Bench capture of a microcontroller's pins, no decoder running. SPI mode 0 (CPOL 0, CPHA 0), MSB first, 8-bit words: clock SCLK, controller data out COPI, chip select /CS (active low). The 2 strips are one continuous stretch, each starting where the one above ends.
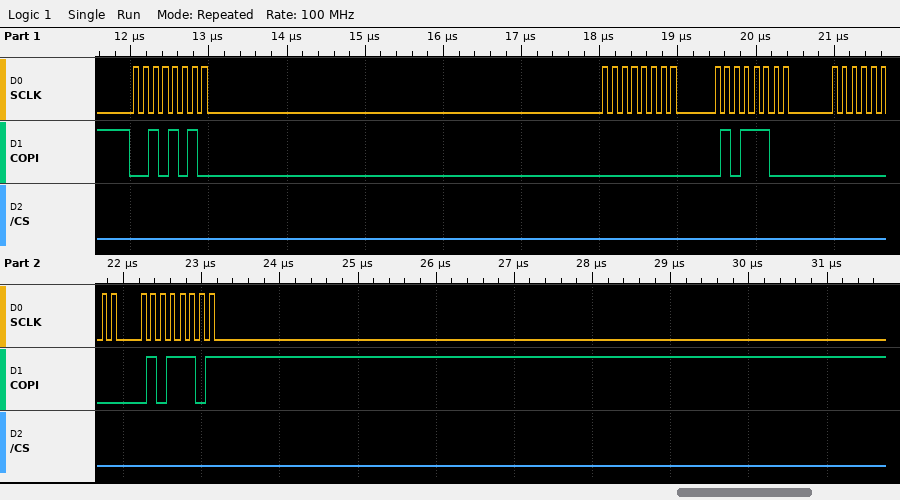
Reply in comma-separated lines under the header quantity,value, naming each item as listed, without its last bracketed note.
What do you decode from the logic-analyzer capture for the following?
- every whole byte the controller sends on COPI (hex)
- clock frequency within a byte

quantity,value
every whole byte the controller sends on COPI,2A 00 5C 00 5D
clock frequency within a byte,8 MHz
